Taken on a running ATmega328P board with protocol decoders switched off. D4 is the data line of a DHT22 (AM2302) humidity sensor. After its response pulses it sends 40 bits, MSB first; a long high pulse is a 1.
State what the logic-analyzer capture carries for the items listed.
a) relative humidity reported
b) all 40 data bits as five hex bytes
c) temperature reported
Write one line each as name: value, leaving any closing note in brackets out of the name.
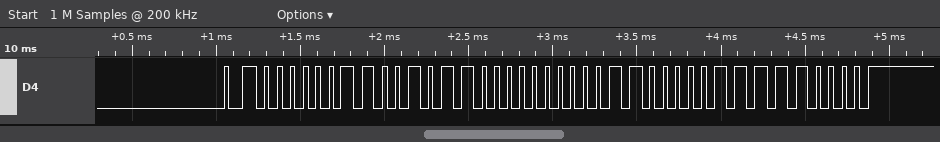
relative humidity reported: 81.2 %
all 40 data bits as five hex bytes: 03 2C 00 C1 F0
temperature reported: 19.3 °C
